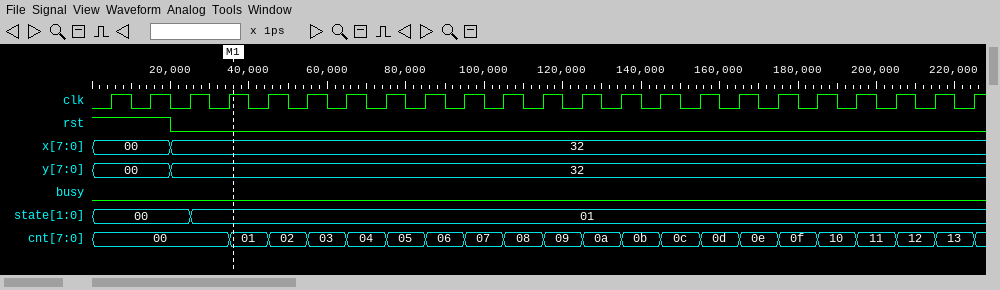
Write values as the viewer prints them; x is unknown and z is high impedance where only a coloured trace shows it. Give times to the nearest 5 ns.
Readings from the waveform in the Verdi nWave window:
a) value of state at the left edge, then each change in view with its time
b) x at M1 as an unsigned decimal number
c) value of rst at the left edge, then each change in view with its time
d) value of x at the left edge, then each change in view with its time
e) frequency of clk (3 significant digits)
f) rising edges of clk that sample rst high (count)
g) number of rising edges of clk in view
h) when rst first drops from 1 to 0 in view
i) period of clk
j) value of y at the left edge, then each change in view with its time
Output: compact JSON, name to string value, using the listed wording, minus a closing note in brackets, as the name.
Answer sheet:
{"value of state at the left edge, then each change in view with its time": "00, 01 at 25 ns", "x at M1 as an unsigned decimal number": "50", "value of rst at the left edge, then each change in view with its time": "1, 0 at 20 ns", "value of x at the left edge, then each change in view with its time": "00, 32 at 20 ns", "frequency of clk": "100 MHz", "rising edges of clk that sample rst high": "2", "number of rising edges of clk in view": "23", "when rst first drops from 1 to 0 in view": "20 ns", "period of clk": "10 ns", "value of y at the left edge, then each change in view with its time": "00, 32 at 20 ns"}
